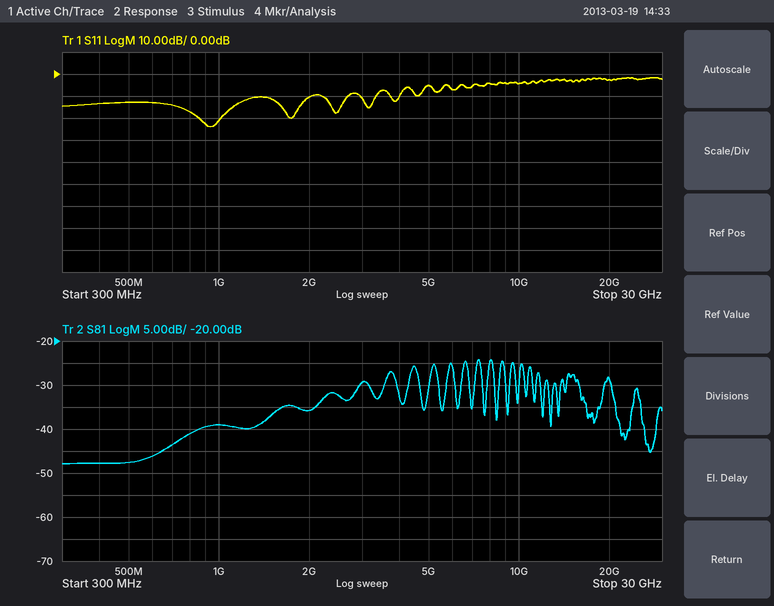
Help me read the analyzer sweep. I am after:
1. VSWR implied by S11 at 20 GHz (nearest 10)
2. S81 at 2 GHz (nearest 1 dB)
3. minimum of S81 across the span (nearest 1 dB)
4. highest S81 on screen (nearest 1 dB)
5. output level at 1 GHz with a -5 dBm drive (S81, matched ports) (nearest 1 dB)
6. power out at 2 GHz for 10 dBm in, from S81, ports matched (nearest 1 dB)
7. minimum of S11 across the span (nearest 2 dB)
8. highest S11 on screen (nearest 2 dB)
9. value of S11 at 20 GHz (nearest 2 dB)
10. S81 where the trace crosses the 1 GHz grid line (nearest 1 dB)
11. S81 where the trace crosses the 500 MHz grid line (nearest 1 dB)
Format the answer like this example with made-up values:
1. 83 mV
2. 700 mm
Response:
1. 10
2. -36 dB
3. -48 dB
4. -24 dB
5. -44 dBm
6. -26 dBm
7. -24 dB
8. -2 dB
9. -2 dB
10. -39 dB
11. -48 dB
